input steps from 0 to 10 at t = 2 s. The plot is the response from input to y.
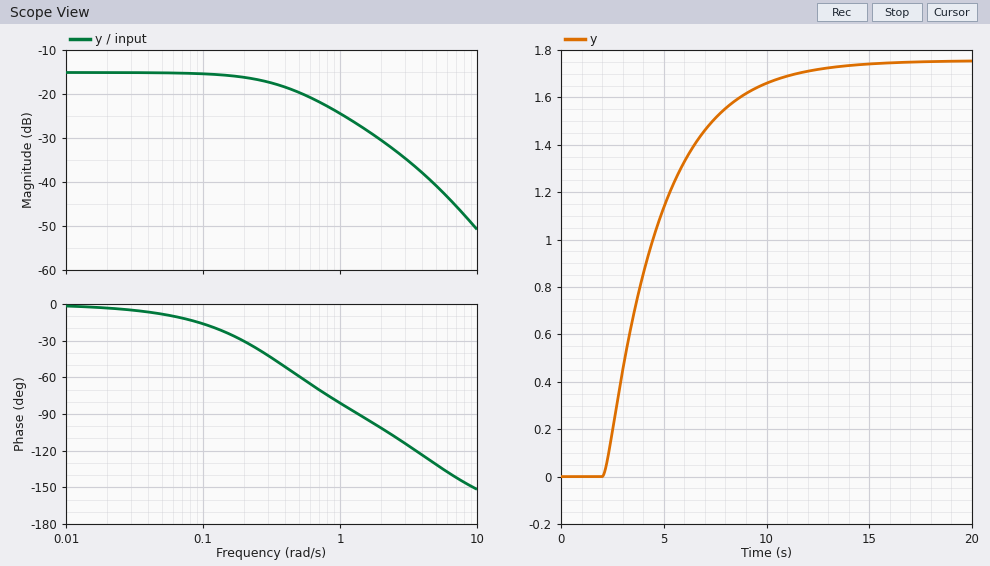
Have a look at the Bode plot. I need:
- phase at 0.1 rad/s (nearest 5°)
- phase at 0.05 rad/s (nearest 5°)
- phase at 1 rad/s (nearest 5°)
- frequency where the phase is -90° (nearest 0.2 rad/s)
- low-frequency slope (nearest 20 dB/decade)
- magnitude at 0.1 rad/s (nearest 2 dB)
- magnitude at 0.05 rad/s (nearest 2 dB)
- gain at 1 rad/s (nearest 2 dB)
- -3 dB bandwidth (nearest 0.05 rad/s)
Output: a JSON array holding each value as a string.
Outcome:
["-15°", "-10°", "-80°", "1.4 rad/s", "0 dB/decade", "-16 dB", "-16 dB", "-24 dB", "0.35 rad/s"]
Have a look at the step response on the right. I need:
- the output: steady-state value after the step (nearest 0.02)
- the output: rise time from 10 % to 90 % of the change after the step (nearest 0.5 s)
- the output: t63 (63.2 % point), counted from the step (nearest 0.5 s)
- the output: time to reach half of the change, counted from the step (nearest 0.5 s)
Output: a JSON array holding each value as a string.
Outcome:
["1.76", "6.0 s", "3.0 s", "2.0 s"]
